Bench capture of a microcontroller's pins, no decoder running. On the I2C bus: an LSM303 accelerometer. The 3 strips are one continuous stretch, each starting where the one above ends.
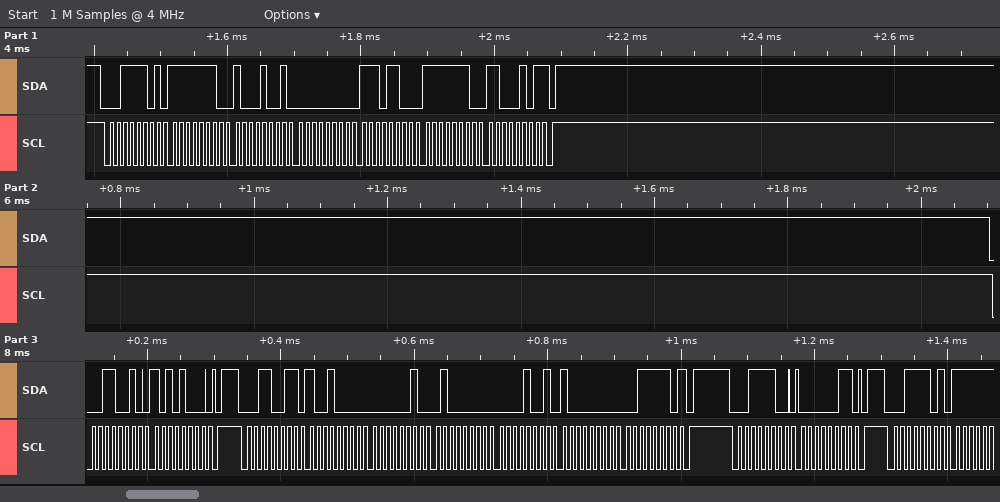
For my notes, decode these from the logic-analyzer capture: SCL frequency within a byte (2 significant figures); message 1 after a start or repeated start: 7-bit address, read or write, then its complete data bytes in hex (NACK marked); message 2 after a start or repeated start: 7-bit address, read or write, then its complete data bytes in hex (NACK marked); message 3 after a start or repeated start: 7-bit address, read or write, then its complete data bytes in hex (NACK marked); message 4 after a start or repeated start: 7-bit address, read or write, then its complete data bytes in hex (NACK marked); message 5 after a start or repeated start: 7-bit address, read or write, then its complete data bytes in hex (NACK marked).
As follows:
100 kHz
0x1E read: FE 89 00 EC FE C5 NACK
0x19 write: A8
0x19 read: 90 02 40 09 80 3E NACK
0x1E write: 03
0x1E read
